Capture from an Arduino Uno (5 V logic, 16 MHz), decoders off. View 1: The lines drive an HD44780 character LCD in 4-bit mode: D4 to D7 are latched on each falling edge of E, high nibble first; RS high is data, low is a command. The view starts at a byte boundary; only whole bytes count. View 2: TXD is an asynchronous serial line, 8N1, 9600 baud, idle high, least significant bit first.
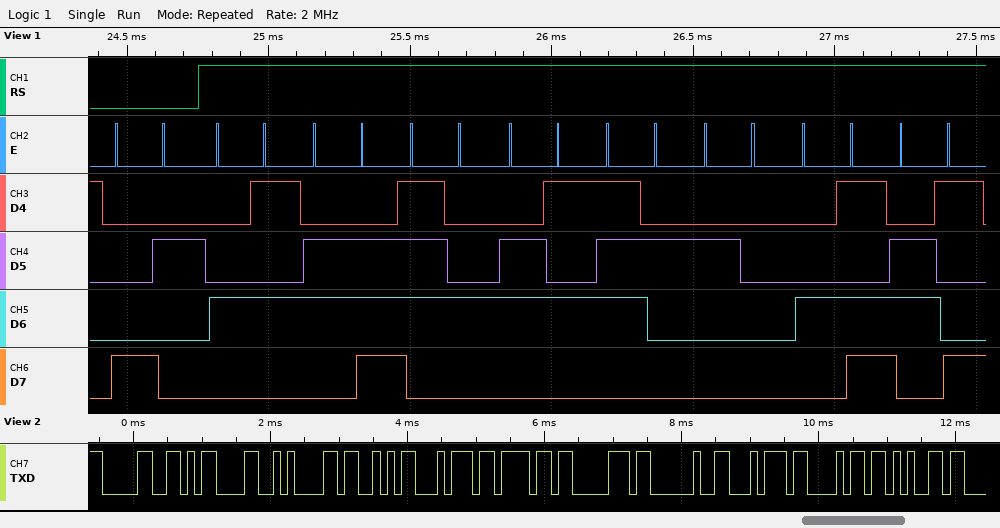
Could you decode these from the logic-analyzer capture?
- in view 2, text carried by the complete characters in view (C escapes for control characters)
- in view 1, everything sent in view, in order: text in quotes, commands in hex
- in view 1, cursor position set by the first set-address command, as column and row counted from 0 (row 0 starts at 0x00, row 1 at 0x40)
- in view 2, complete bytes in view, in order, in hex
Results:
"0\r\nStop the"
0x82 "Enter Mi"
column 2, row 0
30 0D 0A 53 74 6F 70 20 74 68 65
